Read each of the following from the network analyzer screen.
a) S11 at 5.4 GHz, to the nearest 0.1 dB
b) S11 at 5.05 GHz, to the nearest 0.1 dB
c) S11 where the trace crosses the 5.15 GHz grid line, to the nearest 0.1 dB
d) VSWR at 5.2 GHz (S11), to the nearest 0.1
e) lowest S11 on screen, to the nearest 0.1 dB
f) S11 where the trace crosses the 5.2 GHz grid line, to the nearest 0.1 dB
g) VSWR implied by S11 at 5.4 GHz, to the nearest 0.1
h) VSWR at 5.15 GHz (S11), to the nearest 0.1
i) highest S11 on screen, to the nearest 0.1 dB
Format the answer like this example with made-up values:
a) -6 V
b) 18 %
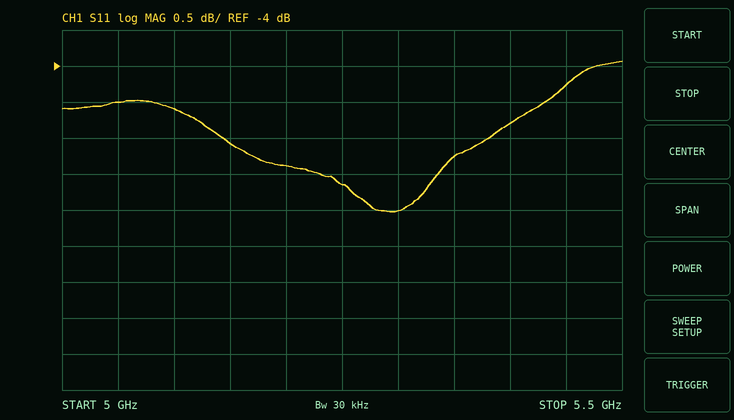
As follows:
a) -4.8 dB
b) -4.5 dB
c) -5.1 dB
d) 3.3
e) -6.0 dB
f) -5.4 dB
g) 3.7
h) 3.5
i) -3.9 dB
